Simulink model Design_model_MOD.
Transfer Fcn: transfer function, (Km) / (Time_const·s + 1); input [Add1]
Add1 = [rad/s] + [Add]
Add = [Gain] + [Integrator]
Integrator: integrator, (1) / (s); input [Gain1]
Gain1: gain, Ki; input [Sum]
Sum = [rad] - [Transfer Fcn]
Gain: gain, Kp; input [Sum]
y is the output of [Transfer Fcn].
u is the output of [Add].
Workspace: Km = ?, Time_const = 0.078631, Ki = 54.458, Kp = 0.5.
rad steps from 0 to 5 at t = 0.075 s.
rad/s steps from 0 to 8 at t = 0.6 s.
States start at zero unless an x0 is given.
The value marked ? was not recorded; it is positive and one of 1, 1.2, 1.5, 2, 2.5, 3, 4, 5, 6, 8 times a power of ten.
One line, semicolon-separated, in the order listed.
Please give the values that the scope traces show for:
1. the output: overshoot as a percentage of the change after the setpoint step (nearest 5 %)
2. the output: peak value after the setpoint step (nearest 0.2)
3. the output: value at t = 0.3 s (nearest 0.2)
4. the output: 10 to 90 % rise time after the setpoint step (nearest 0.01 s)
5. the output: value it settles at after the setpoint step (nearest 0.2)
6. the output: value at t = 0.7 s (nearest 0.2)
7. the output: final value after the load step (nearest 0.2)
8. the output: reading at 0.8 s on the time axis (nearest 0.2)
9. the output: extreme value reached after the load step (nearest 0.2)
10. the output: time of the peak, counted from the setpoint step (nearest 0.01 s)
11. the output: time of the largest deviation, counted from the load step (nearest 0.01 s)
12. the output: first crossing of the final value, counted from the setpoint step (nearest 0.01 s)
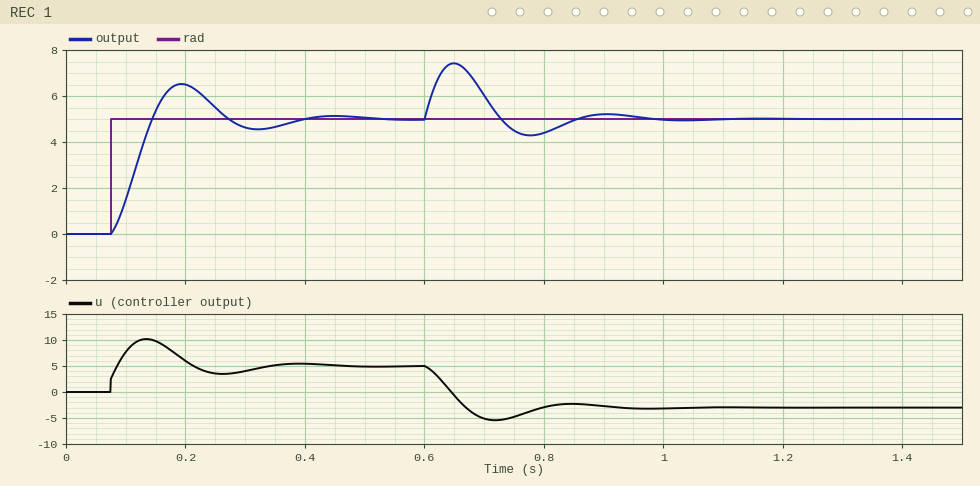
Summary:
30 %; 6.6; 4.6; 0.05 s; 5.0; 6.0; 5.0; 4.4; 7.4; 0.12 s; 0.05 s; 0.07 s
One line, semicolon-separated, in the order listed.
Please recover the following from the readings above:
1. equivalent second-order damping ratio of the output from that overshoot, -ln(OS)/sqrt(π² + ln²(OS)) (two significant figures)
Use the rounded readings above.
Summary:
0.36
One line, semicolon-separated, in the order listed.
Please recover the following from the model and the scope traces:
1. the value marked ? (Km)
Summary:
1
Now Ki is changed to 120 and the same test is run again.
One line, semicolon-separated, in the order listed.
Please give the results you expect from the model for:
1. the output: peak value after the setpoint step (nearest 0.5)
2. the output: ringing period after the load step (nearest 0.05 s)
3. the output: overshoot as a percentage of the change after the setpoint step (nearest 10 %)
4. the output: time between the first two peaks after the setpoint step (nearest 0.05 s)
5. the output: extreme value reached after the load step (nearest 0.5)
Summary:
7.5; 0.15 s; 50 %; 0.15 s; 7.0
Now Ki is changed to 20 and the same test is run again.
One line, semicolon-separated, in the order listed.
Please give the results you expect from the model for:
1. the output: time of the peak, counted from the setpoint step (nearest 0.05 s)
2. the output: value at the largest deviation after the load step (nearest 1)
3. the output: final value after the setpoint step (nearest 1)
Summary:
0.20 s; 8; 5
